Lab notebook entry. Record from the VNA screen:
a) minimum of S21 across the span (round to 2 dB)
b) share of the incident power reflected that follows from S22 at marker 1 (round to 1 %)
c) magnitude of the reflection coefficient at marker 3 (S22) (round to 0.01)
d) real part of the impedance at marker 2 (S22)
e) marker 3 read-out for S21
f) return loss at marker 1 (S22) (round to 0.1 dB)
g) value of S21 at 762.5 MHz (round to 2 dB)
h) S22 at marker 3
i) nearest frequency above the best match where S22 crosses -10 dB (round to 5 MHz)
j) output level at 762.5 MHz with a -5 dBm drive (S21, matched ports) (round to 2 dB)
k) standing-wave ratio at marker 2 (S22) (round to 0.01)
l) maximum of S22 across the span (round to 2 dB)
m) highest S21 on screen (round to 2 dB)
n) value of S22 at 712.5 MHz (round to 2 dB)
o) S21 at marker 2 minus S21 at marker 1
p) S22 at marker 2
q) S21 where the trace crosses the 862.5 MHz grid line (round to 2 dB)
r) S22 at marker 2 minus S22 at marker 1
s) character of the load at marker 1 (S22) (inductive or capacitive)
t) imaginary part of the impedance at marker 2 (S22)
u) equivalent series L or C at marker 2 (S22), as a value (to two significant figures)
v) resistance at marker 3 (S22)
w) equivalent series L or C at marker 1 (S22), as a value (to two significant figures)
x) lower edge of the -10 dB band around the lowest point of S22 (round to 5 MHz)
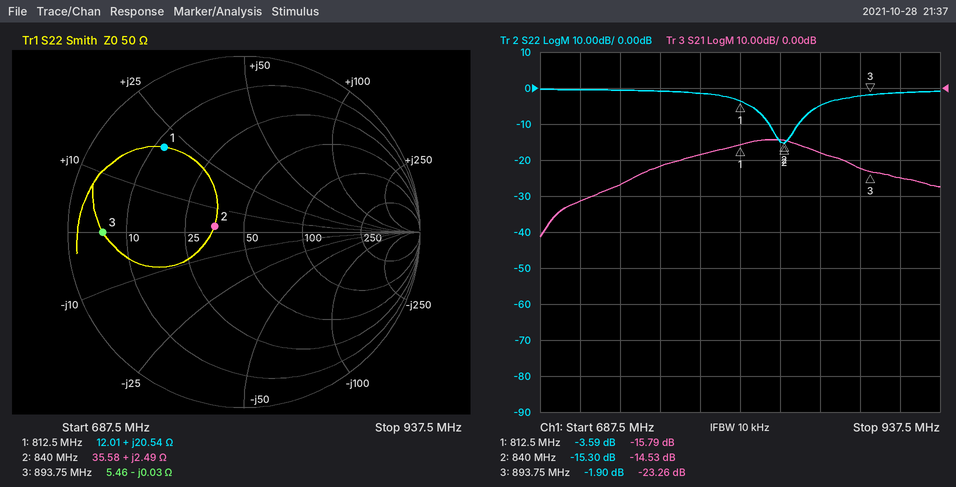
-42 dB
44 %
0.80
35.58 Ω
-23.26 dB
3.6 dB
-22 dB
-1.90 dB
850 MHz
-26 dBm
1.41
0 dB
-14 dB
0 dB
1.26 dB
-15.30 dB
-18 dB
-11.71 dB
inductive
+2.49 Ω
470 pH
5.46 Ω
4.0 nH
830 MHz
